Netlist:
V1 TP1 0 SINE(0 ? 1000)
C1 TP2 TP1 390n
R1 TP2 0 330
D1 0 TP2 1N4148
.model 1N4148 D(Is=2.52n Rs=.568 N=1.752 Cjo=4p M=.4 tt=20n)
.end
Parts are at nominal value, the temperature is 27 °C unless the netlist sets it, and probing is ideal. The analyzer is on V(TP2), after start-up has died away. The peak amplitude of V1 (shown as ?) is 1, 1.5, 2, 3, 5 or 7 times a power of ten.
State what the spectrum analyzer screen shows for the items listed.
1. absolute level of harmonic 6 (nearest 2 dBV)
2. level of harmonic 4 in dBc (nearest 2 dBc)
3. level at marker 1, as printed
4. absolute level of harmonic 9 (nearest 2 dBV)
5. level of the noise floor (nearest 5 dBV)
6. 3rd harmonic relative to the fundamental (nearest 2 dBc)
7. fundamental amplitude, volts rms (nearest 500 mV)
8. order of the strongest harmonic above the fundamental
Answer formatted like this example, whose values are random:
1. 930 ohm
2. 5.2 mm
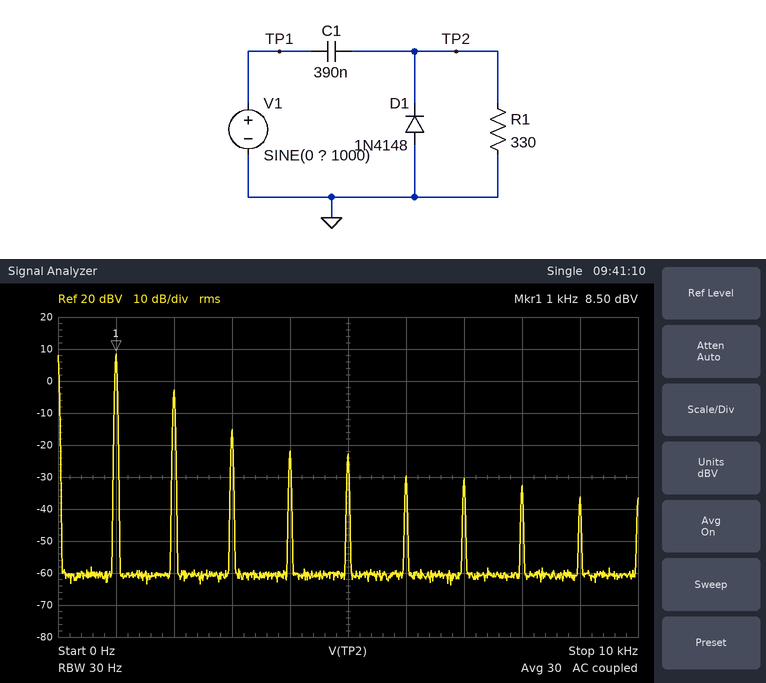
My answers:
1. -30 dBV
2. -30 dBc
3. 8.50 dBV
4. -36 dBV
5. -60 dBV
6. -24 dBc
7. 2.5 V
8. 2
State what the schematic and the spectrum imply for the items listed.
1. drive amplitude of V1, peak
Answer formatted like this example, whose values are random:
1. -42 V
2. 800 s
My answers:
1. 10 V
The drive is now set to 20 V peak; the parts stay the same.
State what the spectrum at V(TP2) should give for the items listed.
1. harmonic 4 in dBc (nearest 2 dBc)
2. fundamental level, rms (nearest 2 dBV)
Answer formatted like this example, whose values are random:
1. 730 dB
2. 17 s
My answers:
1. -28 dBc
2. 14 dBV
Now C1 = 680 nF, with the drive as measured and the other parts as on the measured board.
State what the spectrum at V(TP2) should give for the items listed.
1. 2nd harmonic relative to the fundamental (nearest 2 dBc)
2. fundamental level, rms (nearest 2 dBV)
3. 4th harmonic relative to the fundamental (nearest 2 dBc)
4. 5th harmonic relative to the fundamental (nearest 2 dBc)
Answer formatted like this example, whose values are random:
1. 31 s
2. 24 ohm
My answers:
1. -12 dBc
2. 12 dBV
3. -32 dBc
4. -32 dBc
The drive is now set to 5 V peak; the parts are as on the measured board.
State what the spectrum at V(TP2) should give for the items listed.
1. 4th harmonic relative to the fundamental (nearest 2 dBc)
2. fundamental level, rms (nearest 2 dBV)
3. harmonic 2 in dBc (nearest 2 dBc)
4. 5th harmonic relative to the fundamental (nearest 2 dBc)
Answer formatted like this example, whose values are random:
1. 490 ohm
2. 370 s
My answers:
1. -32 dBc
2. 4 dBV
3. -12 dBc
4. -32 dBc
